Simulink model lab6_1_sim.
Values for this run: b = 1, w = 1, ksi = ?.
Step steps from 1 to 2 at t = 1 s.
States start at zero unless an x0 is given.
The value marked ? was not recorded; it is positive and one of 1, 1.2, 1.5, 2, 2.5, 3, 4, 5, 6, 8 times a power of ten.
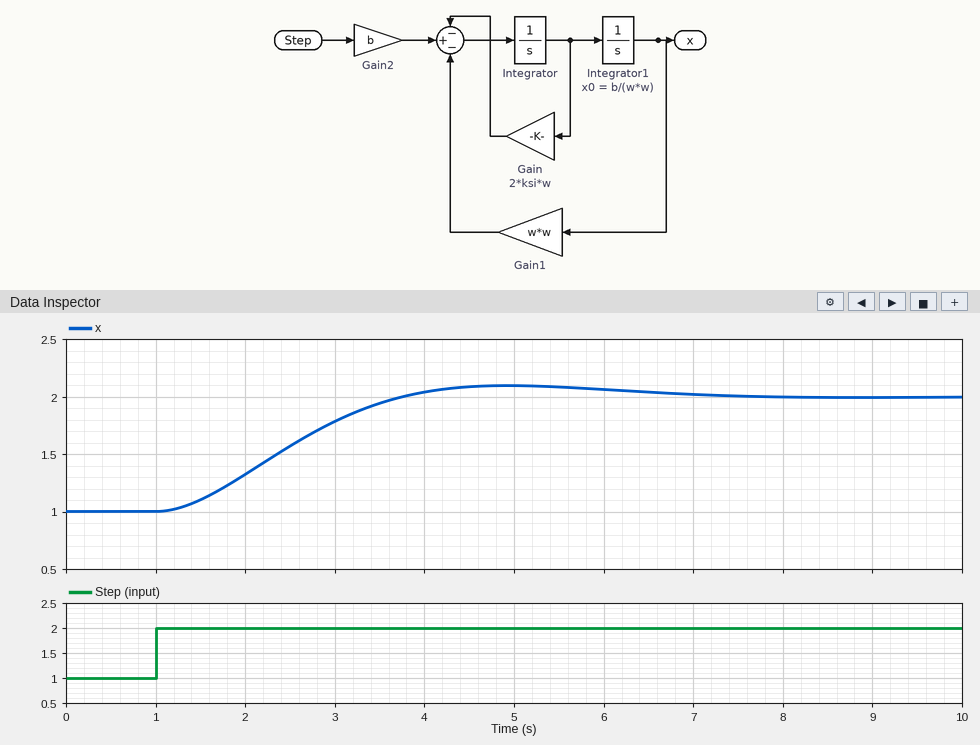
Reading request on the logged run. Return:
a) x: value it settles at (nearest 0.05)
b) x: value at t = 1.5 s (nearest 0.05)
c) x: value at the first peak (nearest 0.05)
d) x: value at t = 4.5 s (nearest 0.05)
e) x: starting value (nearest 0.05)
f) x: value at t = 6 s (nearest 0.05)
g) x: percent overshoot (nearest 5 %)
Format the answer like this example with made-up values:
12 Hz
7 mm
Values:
2.00
1.10
2.10
2.10
1.00
2.05
10 %
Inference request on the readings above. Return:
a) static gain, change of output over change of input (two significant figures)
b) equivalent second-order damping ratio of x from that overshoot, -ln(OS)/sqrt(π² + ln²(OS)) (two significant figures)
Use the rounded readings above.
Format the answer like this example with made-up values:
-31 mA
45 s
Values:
1.0
0.59
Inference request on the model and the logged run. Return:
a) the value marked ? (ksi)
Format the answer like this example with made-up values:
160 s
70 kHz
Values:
0.6
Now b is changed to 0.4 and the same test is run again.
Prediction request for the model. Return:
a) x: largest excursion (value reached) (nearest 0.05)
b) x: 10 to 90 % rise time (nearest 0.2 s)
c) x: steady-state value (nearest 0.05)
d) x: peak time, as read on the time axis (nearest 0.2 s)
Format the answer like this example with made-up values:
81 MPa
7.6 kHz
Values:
0.85
1.8 s
0.80
5.0 s
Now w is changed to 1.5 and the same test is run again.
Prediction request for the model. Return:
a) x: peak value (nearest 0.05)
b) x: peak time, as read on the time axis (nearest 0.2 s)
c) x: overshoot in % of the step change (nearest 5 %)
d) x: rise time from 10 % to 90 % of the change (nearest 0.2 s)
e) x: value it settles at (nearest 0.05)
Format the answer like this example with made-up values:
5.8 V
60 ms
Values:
0.95
3.6 s
10 %
1.2 s
0.90
